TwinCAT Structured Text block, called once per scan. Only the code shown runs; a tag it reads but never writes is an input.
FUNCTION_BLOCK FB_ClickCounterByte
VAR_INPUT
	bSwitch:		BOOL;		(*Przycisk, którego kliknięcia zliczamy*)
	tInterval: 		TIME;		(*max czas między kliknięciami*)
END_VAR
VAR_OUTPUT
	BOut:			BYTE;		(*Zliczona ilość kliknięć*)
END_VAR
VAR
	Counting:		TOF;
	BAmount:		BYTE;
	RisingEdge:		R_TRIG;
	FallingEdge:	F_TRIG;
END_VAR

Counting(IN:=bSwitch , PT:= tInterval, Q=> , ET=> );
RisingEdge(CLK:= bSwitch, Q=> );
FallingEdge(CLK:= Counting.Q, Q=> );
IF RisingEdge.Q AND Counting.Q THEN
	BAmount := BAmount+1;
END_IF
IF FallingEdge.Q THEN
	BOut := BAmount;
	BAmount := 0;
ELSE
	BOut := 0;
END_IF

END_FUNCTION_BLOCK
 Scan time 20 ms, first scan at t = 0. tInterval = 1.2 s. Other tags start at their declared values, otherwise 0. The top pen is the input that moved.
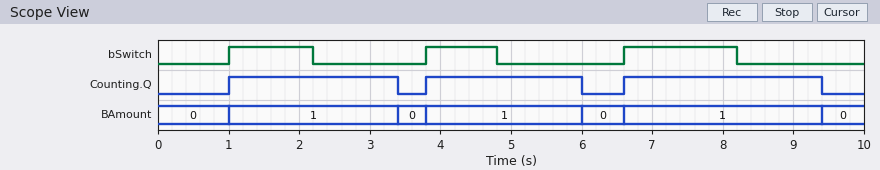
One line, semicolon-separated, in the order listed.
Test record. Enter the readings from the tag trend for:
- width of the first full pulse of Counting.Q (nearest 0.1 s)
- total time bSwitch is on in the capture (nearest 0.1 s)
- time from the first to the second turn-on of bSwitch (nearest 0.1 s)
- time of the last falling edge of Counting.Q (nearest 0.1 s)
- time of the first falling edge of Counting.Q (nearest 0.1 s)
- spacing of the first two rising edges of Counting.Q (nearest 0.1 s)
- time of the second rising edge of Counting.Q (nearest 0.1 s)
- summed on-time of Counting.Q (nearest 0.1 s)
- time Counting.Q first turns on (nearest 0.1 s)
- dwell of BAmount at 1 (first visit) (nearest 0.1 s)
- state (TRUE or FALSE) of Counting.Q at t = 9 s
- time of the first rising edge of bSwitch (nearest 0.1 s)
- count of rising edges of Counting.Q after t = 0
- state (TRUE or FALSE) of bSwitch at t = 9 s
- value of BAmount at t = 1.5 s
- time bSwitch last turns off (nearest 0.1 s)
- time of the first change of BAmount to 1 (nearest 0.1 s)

2.4 s; 3.8 s; 2.8 s; 9.4 s; 3.4 s; 2.8 s; 3.8 s; 7.4 s; 1.0 s; 2.4 s; TRUE; 1.0 s; 3; FALSE; 1; 8.2 s; 1.0 s
